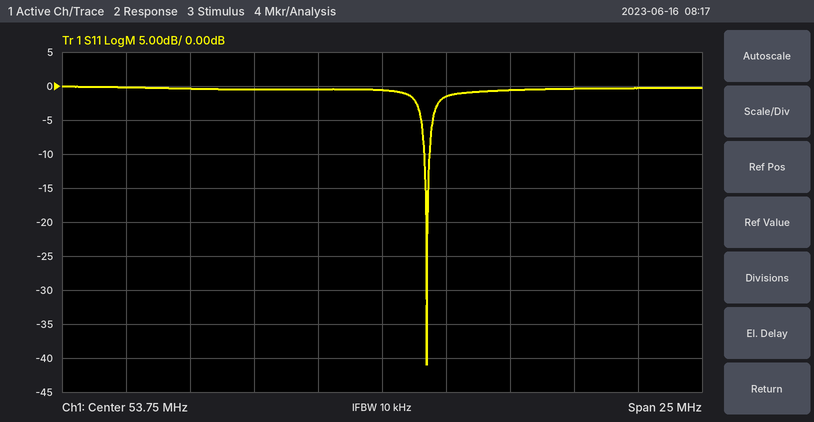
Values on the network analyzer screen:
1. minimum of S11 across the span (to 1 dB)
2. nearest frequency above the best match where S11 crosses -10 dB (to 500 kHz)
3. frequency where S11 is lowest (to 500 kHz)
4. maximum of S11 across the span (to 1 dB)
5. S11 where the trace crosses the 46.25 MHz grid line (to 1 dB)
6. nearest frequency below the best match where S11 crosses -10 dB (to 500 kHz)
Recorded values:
-41 dB
55.5 MHz
55.5 MHz
0 dB
0 dB
55.5 MHz
